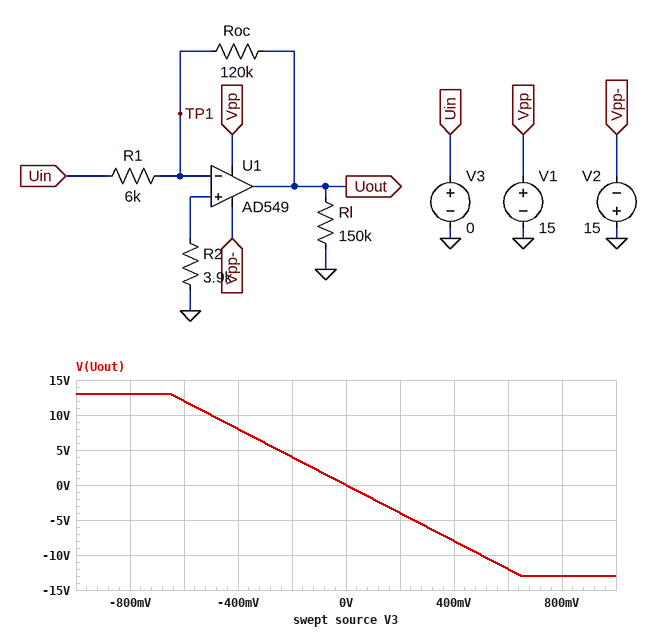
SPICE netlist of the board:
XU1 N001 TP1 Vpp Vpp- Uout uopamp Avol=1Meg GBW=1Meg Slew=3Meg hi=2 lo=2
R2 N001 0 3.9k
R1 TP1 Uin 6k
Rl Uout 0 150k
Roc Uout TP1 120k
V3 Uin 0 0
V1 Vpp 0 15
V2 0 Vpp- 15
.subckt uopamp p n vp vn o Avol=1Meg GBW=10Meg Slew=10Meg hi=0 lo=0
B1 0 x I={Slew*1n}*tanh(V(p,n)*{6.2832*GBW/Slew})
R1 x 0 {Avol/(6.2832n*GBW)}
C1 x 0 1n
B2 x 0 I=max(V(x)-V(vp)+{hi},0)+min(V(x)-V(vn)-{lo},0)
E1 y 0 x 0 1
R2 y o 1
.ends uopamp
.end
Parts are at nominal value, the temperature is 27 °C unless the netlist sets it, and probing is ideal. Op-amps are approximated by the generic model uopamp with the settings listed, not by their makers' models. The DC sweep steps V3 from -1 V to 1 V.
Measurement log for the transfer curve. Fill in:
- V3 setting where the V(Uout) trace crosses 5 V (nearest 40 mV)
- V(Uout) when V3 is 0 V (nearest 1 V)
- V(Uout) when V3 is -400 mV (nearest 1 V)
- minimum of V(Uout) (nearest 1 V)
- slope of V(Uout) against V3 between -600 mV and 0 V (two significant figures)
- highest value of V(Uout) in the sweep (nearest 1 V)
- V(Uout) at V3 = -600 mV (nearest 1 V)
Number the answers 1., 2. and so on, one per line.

1. -240 mV
2. 0 V
3. 8 V
4. -13 V
5. -20 V/V
6. 13 V
7. 12 V
